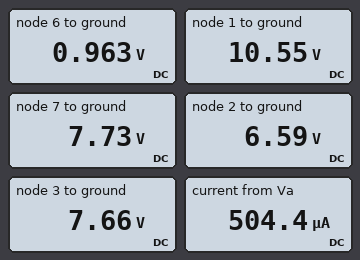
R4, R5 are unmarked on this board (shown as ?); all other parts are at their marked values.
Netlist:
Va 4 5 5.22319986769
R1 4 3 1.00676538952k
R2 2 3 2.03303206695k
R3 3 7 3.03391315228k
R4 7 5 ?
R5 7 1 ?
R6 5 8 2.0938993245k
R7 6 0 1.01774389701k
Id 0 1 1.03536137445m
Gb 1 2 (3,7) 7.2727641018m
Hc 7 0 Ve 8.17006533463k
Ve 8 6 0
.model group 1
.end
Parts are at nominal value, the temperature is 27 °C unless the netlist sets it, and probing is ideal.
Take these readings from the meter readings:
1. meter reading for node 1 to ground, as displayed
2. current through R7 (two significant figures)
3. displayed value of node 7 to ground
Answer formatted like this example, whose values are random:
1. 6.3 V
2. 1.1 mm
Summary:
1. 10.55 V
2. 950 µA
3. 7.73 V
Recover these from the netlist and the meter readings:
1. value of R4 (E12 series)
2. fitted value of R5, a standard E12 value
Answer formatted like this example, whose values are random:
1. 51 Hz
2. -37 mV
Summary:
1. 3.3 kΩ
2. 1.8 kΩ
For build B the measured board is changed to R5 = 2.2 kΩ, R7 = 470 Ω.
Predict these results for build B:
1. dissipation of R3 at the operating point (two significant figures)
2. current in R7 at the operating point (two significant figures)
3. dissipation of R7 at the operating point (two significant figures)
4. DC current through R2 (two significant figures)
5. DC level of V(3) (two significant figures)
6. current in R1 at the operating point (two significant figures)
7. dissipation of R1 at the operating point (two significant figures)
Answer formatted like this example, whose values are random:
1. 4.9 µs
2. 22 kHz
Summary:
1. 2.4 µW
2. 840 µA
3. 330 µW
4. 620 µA
5. 6.8 V
6. 590 µA
7. 350 µW
